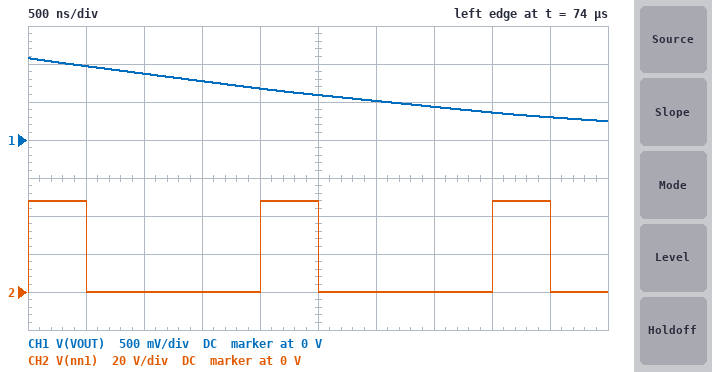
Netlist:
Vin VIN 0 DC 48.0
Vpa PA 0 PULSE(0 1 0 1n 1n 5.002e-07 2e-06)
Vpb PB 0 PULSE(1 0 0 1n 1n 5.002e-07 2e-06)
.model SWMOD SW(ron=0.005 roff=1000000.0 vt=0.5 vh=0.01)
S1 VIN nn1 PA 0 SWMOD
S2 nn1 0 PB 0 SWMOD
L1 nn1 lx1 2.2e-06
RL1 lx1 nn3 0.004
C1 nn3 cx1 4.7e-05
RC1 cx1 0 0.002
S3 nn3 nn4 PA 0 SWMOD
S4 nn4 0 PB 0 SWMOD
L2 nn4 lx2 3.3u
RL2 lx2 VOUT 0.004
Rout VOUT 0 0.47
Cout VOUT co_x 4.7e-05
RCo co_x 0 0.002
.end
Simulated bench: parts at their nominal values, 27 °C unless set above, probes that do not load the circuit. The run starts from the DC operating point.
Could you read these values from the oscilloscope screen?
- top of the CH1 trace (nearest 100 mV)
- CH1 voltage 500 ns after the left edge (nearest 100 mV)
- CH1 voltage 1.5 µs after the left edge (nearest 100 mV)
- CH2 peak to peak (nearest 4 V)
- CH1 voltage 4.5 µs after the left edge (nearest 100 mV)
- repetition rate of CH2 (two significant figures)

1.1 V
1.0 V
800 mV
48 V
300 mV
500 kHz
